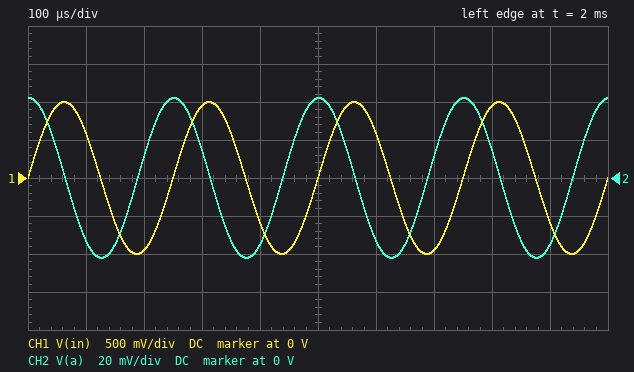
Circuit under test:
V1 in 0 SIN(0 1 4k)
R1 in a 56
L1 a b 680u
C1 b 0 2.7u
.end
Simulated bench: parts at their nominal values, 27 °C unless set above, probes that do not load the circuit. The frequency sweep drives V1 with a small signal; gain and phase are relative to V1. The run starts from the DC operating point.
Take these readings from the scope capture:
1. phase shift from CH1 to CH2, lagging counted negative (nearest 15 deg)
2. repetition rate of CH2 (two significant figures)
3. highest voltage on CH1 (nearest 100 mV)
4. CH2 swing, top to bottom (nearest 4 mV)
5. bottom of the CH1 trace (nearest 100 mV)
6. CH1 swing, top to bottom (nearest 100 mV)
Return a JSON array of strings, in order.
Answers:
["90 deg", "4.0 kHz", "1.0 V", "84 mV", "-1.0 V", "2.0 V"]
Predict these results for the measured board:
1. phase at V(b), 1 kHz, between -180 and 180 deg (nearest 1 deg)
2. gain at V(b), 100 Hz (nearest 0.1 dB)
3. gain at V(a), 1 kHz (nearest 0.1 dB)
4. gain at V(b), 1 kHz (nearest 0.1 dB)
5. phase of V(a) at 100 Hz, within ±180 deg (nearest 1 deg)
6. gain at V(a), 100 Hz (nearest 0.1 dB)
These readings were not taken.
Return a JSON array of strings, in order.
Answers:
["-46 deg", "0 dB", "-3.1 dB", "-2.5 dB", "-5 deg", "0 dB"]
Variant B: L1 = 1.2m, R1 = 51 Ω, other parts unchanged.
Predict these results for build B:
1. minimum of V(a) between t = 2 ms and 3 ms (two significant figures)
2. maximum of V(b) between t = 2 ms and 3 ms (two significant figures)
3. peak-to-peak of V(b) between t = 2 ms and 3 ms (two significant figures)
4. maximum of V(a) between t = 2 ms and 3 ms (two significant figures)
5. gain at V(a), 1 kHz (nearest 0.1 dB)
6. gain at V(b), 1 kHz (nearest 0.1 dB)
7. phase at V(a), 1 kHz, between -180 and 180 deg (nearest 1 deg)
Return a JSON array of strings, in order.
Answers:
["-290 mV", "280 mV", "550 mV", "290 mV", "-3.0 dB", "-1.8 dB", "-45 deg"]
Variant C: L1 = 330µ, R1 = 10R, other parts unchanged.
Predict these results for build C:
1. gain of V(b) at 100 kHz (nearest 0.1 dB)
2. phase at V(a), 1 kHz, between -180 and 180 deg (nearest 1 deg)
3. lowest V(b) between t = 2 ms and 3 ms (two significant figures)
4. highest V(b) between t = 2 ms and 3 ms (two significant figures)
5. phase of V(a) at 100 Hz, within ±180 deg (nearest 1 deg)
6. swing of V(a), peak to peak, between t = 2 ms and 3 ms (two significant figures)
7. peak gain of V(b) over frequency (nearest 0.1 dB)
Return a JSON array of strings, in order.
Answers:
["-50.9 dB", "-10 deg", "-1.2 V", "1.2 V", "-1 deg", "1.1 V", "1.9 dB"]
